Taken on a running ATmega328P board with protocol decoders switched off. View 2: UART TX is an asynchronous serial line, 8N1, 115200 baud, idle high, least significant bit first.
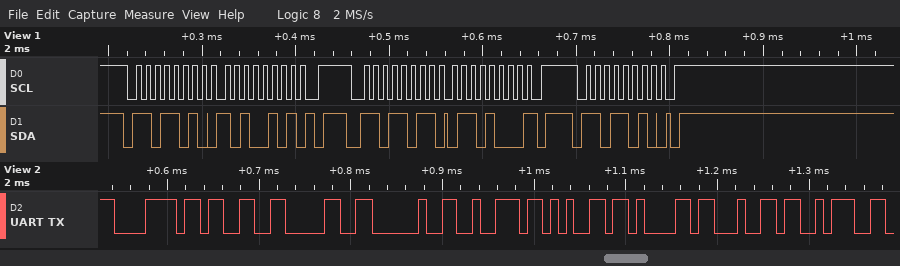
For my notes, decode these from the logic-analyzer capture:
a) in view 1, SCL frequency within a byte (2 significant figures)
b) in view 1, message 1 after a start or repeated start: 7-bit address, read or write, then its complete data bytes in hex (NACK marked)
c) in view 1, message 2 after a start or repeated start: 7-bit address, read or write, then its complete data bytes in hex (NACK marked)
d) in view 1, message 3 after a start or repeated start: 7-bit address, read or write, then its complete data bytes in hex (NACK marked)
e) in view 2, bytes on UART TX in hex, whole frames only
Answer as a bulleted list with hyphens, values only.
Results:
- 100 kHz
- 0x6D write: A5
- 0x6D read: 68 NACK
- 0x6D write
- 0x78 0x33 0x30 0x20 0x72 0x65 0x61 0x64 0x3A
